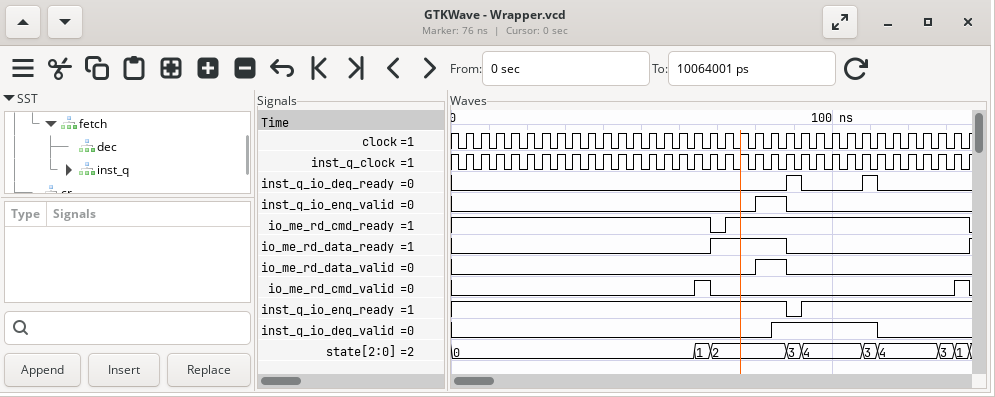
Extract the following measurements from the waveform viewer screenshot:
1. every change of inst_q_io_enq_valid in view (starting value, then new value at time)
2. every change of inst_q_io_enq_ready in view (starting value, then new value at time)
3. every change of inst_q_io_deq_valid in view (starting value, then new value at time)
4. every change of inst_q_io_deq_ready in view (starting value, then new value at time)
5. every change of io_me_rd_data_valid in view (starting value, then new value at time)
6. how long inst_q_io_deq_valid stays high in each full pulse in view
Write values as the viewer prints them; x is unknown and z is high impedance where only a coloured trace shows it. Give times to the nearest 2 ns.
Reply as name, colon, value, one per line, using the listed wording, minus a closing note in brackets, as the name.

every change of inst_q_io_enq_valid in view: 0, 1 at 80 ns, 0 at 88 ns
every change of inst_q_io_enq_ready in view: 1, 0 at 88 ns, 1 at 92 ns
every change of inst_q_io_deq_valid in view: 0, 1 at 84 ns, 0 at 112 ns
every change of inst_q_io_deq_ready in view: 0, 1 at 88 ns, 0 at 92 ns, 1 at 108 ns, 0 at 112 ns
every change of io_me_rd_data_valid in view: 0, 1 at 80 ns, 0 at 88 ns
how long inst_q_io_deq_valid stays high in each full pulse in view: 28 ns
